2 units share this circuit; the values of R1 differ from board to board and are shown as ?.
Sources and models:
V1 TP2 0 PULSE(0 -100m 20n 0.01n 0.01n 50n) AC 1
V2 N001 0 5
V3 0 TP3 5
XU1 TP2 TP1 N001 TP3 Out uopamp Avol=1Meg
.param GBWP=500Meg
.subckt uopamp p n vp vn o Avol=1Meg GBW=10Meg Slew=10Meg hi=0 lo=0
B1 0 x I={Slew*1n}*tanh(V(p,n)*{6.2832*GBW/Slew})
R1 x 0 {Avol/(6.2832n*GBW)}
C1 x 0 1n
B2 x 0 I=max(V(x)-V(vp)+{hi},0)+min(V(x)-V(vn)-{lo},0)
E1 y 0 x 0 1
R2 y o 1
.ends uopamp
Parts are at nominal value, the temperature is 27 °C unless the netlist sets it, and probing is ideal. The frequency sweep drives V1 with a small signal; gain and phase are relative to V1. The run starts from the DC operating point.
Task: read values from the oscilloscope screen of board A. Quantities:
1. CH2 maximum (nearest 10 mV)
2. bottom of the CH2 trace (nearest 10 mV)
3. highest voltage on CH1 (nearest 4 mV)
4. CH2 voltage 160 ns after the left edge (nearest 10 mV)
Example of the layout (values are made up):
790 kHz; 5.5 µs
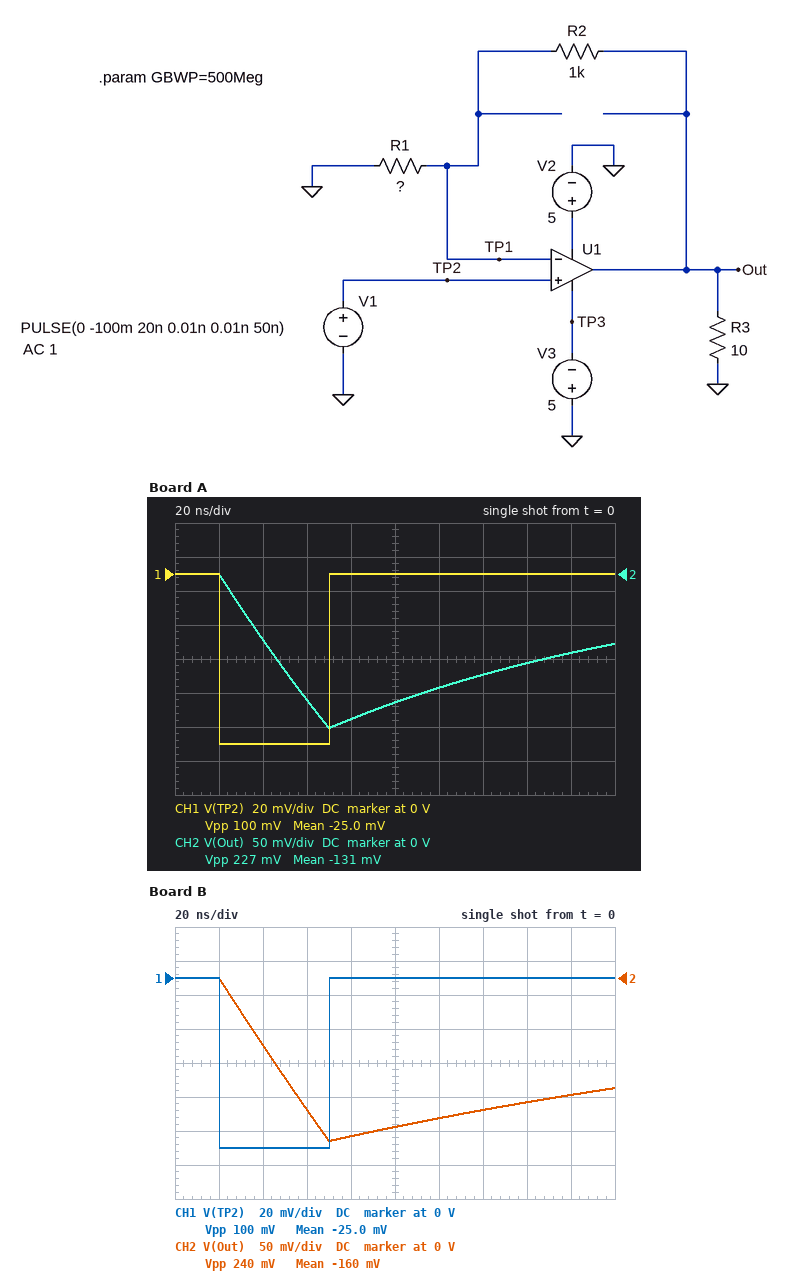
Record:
0 V; -230 mV; 0 V; -130 mV
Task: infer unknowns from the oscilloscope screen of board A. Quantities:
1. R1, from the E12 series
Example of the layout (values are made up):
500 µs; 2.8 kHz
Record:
120 Ω
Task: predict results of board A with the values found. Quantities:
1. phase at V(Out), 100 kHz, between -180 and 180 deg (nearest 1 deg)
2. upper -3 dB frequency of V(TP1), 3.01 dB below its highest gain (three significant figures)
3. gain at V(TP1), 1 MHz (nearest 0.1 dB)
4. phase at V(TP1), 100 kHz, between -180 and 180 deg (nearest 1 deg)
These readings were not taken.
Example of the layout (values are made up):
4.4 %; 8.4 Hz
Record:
-6 deg; 973 kHz; -3.1 dB; -6 deg
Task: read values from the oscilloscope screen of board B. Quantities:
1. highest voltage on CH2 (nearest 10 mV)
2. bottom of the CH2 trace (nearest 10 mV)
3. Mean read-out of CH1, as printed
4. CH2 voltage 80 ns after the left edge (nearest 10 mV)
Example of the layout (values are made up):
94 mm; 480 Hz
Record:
0 V; -240 mV; -25.0 mV; -230 mV
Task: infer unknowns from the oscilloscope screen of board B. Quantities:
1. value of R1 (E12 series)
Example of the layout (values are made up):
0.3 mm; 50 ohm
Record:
56 Ω
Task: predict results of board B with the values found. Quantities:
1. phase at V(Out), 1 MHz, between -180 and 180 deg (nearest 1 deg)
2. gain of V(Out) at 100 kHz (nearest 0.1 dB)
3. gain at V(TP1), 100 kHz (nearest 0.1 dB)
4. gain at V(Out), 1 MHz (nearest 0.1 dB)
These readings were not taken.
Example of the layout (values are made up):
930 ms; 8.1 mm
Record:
-64 deg; 25.3 dB; -0.2 dB; 18.3 dB
